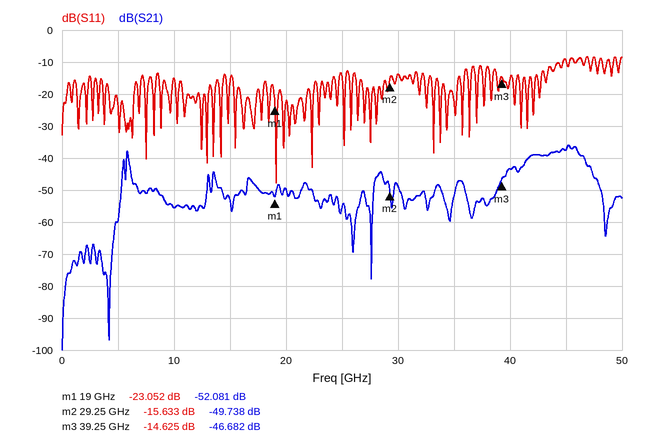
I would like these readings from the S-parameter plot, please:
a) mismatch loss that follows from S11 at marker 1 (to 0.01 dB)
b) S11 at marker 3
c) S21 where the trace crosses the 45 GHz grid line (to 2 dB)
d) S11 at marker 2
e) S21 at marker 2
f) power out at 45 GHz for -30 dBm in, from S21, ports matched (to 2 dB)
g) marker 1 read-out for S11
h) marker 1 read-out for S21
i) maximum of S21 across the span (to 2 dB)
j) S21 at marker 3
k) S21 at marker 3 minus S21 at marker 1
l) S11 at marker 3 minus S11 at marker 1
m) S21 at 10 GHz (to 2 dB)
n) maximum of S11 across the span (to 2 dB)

0.02 dB
-14.625 dB
-38 dB
-15.633 dB
-49.738 dB
-68 dBm
-23.052 dB
-52.081 dB
-36 dB
-46.682 dB
5.399 dB
8.427 dB
-56 dB
-8 dB
